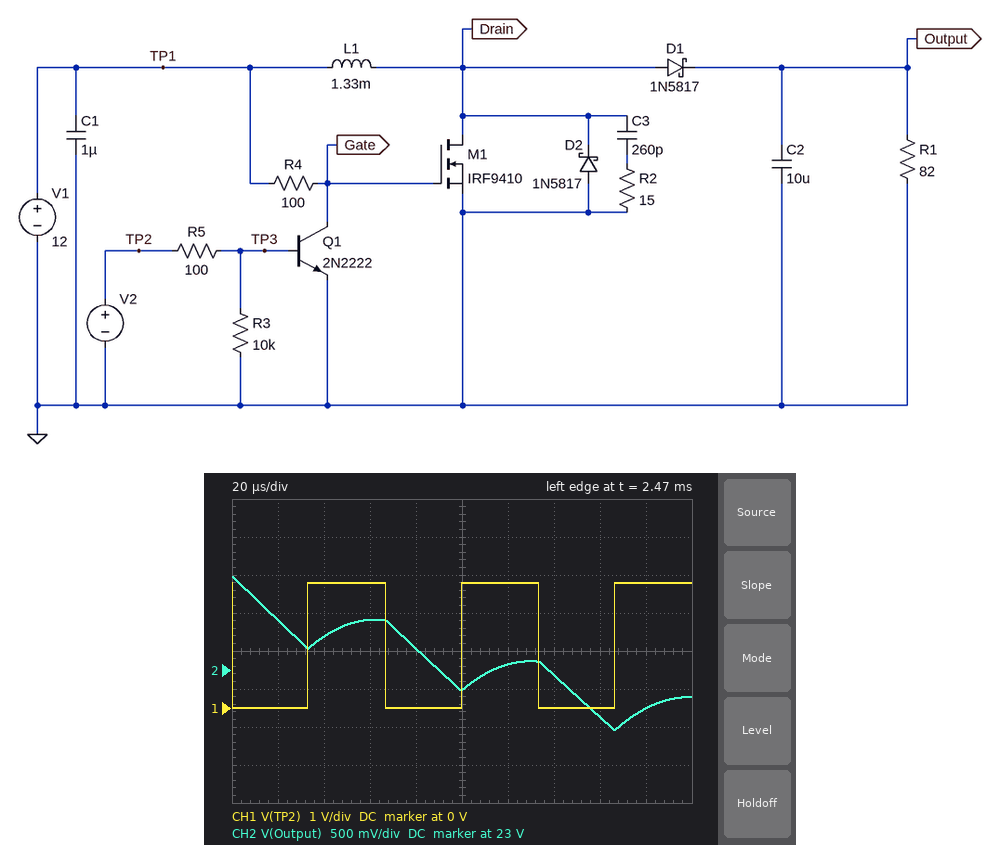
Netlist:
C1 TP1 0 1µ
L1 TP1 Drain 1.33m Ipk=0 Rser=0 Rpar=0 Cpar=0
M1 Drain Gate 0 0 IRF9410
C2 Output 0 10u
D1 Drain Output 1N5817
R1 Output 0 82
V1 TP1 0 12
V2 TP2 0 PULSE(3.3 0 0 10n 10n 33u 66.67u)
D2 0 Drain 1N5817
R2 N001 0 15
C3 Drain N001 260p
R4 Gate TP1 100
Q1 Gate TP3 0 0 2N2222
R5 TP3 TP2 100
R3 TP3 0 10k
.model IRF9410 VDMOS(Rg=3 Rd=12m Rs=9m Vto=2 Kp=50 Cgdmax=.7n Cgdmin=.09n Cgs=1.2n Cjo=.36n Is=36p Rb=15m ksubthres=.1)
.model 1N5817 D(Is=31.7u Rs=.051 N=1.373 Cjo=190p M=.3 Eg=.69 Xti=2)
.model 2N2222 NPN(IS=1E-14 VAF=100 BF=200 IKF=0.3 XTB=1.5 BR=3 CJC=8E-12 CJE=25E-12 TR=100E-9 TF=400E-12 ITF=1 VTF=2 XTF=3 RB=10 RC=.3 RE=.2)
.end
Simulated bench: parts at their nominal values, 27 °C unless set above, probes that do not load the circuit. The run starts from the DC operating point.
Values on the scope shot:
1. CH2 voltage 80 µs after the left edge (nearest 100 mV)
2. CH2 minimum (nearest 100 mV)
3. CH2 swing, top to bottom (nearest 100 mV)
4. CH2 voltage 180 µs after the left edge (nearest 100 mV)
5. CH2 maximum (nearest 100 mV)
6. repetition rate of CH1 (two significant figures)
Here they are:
23.3 V
22.2 V
2.0 V
22.5 V
24.2 V
15 kHz
